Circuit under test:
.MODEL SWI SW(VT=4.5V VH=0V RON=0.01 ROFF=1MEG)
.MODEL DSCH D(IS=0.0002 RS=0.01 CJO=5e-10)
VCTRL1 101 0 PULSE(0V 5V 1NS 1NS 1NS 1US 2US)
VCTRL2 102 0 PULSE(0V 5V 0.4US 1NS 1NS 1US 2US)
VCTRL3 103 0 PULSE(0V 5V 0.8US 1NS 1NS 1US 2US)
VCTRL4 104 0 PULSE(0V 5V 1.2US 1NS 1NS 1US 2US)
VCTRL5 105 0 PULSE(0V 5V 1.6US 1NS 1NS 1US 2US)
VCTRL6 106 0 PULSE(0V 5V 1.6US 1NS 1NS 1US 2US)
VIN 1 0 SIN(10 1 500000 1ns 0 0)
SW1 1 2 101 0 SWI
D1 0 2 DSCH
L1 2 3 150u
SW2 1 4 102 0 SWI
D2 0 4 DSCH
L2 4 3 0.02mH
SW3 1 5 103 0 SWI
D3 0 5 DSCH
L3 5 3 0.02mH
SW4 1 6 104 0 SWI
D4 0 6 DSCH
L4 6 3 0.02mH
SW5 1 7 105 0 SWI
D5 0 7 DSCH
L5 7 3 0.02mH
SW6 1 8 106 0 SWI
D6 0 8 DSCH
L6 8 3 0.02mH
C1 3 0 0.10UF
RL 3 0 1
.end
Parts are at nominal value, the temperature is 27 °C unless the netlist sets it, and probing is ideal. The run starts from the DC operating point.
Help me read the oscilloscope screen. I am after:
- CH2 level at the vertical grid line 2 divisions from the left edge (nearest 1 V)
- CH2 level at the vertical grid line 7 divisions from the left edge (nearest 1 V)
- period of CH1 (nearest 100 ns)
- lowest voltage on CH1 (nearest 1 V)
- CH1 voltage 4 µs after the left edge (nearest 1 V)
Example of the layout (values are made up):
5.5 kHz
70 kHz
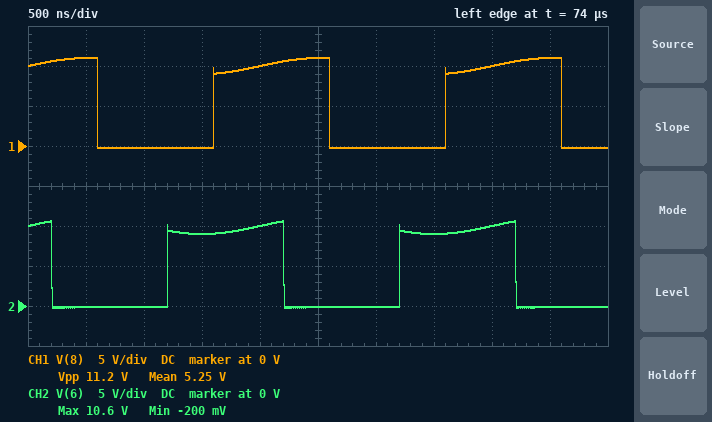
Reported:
0 V
9 V
2.0 µs
0 V
10 V
